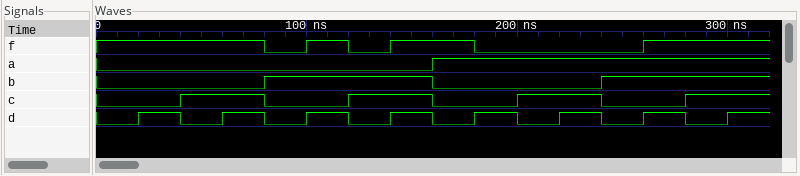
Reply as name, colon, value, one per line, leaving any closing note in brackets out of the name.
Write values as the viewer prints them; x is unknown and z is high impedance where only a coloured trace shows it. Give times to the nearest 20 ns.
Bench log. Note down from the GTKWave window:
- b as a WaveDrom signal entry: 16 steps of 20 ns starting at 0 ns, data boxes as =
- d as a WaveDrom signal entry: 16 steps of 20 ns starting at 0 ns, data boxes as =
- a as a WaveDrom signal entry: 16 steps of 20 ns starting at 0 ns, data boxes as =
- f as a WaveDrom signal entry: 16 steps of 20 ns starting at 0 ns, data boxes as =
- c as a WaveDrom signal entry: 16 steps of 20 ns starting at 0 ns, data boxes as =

b as a WaveDrom signal entry: 16 steps of 20 ns starting at 0 ns, data boxes as =: {name: 'b', wave: '0...1...0...1...'}
d as a WaveDrom signal entry: 16 steps of 20 ns starting at 0 ns, data boxes as =: {name: 'd', wave: '0101010101010101'}
a as a WaveDrom signal entry: 16 steps of 20 ns starting at 0 ns, data boxes as =: {name: 'a', wave: '0.......1.......'}
f as a WaveDrom signal entry: 16 steps of 20 ns starting at 0 ns, data boxes as =: {name: 'f', wave: '1...0101.0...1..'}
c as a WaveDrom signal entry: 16 steps of 20 ns starting at 0 ns, data boxes as =: {name: 'c', wave: '0.1.0.1.0.1.0.1.'}
